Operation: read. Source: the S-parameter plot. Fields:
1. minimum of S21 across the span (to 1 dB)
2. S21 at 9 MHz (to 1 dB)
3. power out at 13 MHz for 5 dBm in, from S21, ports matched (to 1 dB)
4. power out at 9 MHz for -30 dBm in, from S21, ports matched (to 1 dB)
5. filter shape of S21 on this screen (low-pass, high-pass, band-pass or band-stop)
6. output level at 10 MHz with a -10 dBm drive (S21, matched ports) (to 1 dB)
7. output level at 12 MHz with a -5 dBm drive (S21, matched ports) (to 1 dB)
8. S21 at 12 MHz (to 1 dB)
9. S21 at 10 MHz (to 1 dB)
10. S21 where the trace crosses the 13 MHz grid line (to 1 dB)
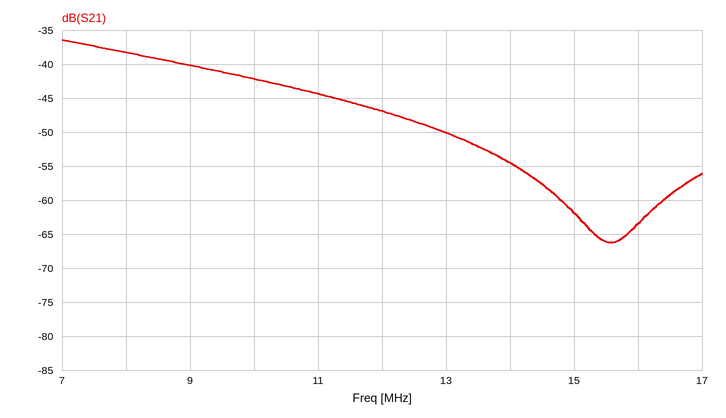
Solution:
-66 dB
-40 dB
-45 dBm
-70 dBm
low-pass
-52 dBm
-52 dBm
-47 dB
-42 dB
-50 dB
